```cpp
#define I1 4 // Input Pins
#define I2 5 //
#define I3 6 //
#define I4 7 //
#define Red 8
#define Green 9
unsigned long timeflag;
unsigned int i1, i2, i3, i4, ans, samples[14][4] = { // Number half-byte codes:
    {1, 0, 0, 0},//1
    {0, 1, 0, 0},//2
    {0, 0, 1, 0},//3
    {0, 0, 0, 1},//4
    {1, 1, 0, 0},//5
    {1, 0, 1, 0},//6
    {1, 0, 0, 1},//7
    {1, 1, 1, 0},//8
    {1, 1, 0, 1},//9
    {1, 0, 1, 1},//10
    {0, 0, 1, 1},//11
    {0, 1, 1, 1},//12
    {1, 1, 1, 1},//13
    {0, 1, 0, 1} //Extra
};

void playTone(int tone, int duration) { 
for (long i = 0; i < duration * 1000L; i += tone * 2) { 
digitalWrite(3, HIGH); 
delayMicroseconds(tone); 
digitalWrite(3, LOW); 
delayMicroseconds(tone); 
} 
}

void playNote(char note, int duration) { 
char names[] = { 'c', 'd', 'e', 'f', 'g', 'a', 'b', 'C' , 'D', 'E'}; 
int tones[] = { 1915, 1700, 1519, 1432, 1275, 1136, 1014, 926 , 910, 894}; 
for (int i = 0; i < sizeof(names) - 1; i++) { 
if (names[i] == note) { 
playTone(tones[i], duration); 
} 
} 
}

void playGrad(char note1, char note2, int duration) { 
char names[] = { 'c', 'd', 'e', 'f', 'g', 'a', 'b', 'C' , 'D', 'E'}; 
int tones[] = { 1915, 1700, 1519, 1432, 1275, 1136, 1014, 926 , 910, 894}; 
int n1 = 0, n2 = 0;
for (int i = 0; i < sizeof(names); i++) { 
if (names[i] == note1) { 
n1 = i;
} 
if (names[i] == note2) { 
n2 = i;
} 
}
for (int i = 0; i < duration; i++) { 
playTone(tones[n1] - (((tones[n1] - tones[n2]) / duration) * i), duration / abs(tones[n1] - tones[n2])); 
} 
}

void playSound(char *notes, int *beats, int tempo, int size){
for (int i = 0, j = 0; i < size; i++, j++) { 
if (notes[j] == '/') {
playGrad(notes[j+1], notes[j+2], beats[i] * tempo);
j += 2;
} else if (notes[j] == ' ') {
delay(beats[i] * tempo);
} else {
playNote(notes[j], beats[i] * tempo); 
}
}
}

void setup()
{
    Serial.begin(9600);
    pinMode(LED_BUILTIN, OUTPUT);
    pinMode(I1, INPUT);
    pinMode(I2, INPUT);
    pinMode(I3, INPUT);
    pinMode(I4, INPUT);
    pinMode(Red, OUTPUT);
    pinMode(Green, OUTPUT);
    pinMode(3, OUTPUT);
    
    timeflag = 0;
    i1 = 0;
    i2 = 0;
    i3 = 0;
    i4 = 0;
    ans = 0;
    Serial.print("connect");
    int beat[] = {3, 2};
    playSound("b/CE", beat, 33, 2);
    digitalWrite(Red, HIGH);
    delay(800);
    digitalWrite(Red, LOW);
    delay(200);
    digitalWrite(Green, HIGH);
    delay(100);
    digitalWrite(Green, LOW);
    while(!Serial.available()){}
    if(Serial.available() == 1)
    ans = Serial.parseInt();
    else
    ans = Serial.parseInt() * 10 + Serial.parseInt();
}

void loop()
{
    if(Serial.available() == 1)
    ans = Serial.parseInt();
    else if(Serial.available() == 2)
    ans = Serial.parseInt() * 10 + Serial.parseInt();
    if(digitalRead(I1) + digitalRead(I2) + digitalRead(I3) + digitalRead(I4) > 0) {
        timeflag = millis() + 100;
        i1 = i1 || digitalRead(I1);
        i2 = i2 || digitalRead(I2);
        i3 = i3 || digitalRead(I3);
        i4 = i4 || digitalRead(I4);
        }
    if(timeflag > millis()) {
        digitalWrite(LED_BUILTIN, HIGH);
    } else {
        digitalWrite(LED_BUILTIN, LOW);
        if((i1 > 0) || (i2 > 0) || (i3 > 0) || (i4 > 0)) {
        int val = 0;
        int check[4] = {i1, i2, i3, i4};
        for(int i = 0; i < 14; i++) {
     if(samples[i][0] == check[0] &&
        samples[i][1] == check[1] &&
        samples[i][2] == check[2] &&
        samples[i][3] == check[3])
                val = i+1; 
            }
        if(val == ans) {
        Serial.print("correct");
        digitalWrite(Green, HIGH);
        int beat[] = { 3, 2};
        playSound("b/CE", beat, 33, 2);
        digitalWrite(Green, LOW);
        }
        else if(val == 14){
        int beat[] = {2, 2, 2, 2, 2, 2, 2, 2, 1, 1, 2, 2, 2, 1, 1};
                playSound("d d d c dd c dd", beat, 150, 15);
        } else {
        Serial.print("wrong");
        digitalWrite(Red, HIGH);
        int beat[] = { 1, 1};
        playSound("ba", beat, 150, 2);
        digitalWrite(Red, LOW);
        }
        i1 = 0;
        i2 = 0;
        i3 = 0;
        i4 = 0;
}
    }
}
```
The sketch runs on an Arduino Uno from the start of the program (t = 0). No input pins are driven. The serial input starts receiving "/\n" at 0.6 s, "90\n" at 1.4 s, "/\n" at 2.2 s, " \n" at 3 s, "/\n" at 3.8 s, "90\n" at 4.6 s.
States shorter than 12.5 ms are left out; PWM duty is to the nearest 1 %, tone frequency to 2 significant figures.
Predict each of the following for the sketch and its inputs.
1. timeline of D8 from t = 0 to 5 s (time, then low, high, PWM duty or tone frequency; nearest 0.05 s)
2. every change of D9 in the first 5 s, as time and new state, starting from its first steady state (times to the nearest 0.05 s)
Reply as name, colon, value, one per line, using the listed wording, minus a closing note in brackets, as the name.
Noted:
timeline of D8 from t = 0 to 5 s: 0 s low; 0.35 s high; 1.15 s low
every change of D9 in the first 5 s, as time and new state, starting from its first steady state: 0 s low; 1.35 s high; 1.45 s low
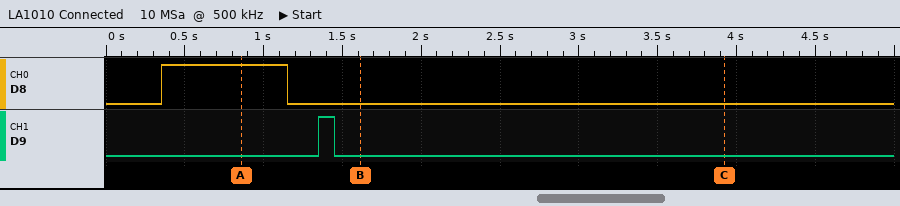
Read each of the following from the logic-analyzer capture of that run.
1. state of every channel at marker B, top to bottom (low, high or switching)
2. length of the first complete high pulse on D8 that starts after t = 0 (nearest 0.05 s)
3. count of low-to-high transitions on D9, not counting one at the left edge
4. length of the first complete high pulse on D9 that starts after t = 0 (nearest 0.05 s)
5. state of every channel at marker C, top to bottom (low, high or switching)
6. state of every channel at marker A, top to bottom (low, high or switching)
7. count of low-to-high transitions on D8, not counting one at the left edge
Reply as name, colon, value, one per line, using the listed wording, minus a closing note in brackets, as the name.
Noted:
state of every channel at marker B, top to bottom: D8 low, D9 low
length of the first complete high pulse on D8 that starts after t = 0: 0.80 s
count of low-to-high transitions on D9, not counting one at the left edge: 1
length of the first complete high pulse on D9 that starts after t = 0: 0.10 s
state of every channel at marker C, top to bottom: D8 low, D9 low
state of every channel at marker A, top to bottom: D8 high, D9 low
count of low-to-high transitions on D8, not counting one at the left edge: 1
